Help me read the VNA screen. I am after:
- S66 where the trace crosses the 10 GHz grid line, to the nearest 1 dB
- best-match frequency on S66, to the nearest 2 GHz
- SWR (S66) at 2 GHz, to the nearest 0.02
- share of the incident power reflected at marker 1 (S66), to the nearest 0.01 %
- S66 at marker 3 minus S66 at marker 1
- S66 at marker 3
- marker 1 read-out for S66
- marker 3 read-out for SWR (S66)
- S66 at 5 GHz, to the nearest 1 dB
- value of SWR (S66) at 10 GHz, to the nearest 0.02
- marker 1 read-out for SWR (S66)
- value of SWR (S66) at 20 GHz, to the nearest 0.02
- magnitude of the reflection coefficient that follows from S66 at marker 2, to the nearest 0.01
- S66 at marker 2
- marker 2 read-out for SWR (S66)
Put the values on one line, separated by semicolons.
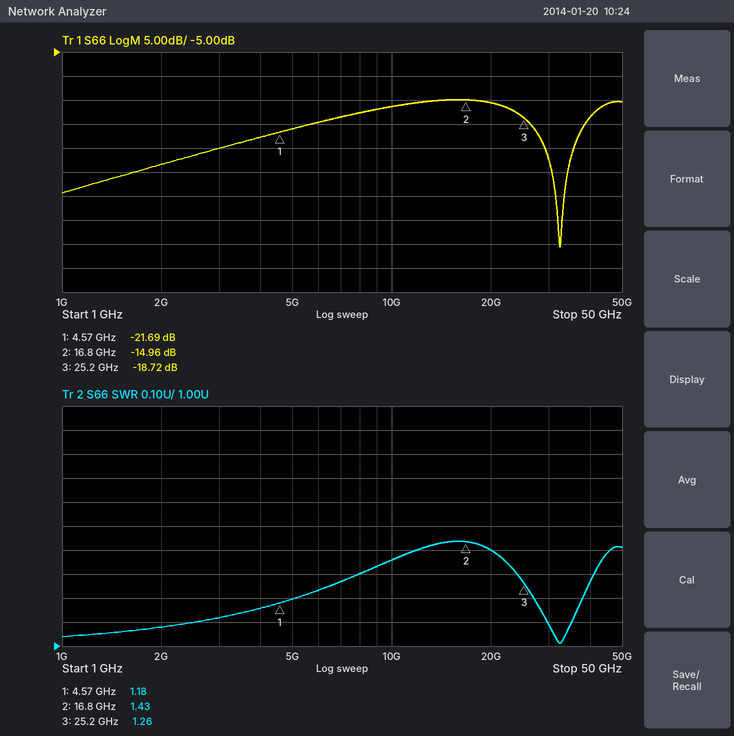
-16 dB; 32 GHz; 1.08; 0.68 %; 2.97 dB; -18.72 dB; -21.69 dB; 1.26; -21 dB; 1.36; 1.18; 1.40; 0.18; -14.96 dB; 1.43
